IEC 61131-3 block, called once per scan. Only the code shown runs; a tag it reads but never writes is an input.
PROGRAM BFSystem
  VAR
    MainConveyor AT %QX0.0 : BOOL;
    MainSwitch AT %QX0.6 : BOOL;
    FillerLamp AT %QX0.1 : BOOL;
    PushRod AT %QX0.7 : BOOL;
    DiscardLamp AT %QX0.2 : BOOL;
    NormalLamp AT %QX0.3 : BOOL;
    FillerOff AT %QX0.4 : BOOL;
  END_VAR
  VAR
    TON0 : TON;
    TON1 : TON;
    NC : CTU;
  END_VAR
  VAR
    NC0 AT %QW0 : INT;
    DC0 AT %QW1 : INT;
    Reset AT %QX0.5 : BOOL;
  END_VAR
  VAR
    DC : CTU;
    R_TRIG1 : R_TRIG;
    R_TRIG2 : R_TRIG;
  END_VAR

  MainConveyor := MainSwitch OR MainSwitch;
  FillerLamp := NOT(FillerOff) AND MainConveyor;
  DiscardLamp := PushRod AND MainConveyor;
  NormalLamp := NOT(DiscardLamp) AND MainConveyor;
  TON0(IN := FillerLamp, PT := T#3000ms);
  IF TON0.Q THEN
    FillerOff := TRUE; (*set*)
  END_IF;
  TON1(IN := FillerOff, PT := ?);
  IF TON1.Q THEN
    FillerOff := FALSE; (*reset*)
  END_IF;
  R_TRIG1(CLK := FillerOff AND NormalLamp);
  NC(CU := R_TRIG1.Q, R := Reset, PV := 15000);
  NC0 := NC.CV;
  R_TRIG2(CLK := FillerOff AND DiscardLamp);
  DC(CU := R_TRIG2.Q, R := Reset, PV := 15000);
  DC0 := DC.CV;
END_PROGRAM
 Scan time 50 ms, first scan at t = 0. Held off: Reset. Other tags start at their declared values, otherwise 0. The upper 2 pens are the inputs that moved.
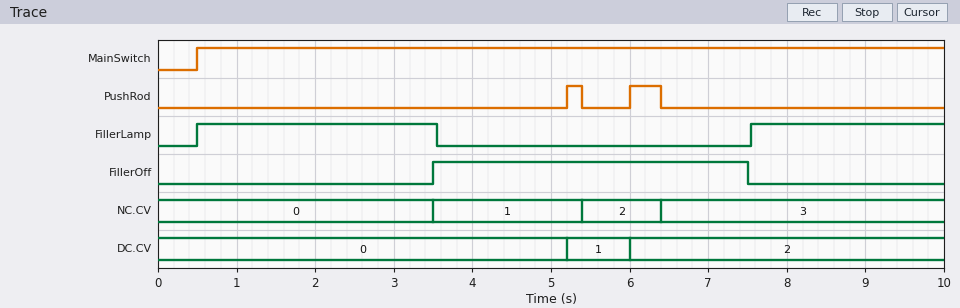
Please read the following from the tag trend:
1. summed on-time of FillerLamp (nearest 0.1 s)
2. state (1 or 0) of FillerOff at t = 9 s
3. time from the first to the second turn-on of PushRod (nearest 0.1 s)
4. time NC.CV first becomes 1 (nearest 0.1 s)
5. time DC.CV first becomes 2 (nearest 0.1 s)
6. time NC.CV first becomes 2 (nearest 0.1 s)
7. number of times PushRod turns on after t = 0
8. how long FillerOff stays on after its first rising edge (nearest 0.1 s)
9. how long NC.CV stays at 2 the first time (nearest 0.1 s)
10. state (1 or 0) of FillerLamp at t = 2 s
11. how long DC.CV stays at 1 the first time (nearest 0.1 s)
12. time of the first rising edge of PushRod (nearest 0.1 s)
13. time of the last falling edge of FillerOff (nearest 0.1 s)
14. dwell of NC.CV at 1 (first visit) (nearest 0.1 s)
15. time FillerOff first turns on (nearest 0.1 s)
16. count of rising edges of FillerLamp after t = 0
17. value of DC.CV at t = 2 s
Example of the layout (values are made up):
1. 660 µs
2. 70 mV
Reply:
1. 5.5 s
2. 0
3. 0.8 s
4. 3.5 s
5. 6.0 s
6. 5.4 s
7. 2
8. 4.0 s
9. 1.0 s
10. 1
11. 0.8 s
12. 5.2 s
13. 7.5 s
14. 1.9 s
15. 3.5 s
16. 2
17. 0
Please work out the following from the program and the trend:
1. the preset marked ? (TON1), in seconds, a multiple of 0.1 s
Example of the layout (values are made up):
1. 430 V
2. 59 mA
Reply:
1. 4.0 s
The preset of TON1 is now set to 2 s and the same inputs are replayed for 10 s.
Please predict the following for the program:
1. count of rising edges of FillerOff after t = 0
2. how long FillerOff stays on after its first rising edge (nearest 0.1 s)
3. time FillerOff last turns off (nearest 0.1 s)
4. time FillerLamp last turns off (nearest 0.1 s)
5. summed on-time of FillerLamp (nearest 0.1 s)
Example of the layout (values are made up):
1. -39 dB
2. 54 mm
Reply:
1. 2
2. 2.0 s
3. 5.5 s
4. 8.6 s
5. 6.1 s
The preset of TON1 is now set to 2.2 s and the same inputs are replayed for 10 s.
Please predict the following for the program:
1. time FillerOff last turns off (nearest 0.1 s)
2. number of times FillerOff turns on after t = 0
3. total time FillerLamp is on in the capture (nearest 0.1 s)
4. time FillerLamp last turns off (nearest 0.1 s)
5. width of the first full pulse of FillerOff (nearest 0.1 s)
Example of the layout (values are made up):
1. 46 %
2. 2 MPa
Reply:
1. 5.7 s
2. 2
3. 6.1 s
4. 8.8 s
5. 2.2 s
